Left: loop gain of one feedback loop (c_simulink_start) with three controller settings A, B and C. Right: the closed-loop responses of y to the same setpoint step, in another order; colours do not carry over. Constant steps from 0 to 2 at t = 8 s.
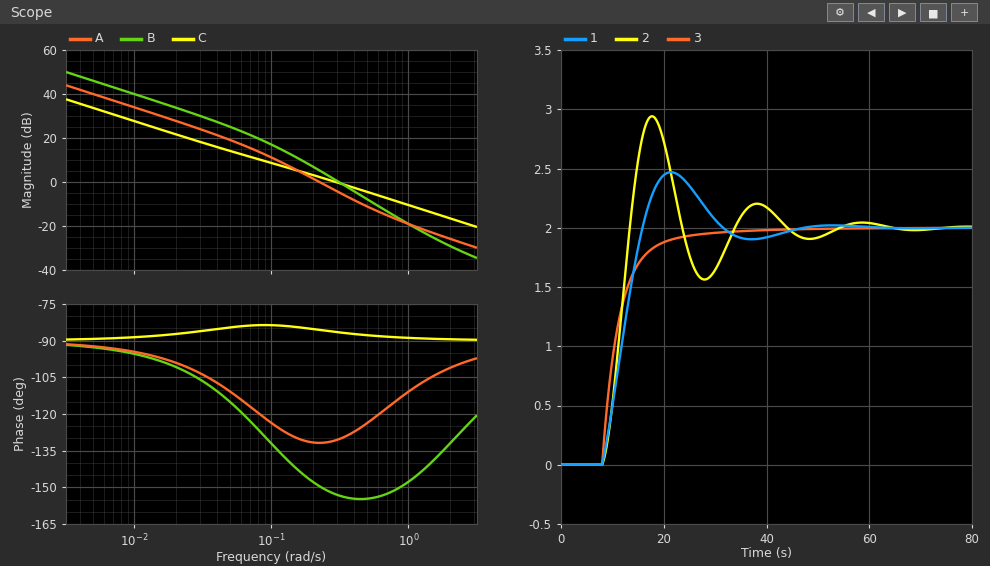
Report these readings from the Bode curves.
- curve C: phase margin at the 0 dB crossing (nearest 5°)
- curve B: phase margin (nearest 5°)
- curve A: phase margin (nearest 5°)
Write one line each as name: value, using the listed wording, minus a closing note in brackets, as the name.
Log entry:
curve C: phase margin at the 0 dB crossing: 95°
curve B: phase margin: 25°
curve A: phase margin: 50°
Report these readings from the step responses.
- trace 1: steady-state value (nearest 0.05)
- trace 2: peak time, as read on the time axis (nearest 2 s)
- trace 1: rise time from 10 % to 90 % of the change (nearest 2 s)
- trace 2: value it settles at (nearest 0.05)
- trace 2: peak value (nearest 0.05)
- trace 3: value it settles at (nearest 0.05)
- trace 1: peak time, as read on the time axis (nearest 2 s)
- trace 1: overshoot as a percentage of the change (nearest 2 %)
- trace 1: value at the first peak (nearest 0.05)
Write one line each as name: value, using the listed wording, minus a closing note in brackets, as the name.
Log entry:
trace 1: steady-state value: 2.00
trace 2: peak time, as read on the time axis: 18 s
trace 1: rise time from 10 % to 90 % of the change: 6 s
trace 2: value it settles at: 2.00
trace 2: peak value: 2.95
trace 3: value it settles at: 2.00
trace 1: peak time, as read on the time axis: 22 s
trace 1: overshoot as a percentage of the change: 24 %
trace 1: value at the first peak: 2.45
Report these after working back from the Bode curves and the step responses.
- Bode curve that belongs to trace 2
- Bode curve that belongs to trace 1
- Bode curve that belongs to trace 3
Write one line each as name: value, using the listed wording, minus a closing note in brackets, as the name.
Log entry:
Bode curve that belongs to trace 2: B
Bode curve that belongs to trace 1: A
Bode curve that belongs to trace 3: C
